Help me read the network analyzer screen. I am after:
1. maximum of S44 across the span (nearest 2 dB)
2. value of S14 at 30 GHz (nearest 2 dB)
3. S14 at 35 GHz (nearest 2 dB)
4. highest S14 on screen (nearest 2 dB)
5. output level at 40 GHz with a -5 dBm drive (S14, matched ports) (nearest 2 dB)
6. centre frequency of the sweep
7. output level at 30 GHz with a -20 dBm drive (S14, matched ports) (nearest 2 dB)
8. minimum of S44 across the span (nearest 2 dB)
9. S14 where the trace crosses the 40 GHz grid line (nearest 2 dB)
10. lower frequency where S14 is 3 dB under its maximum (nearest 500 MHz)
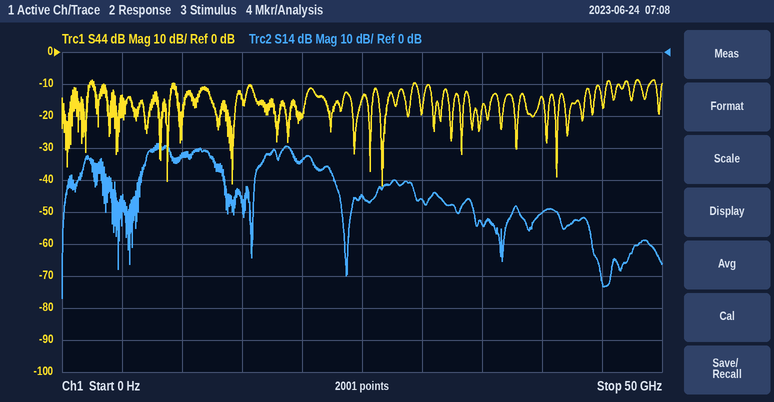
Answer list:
-8 dB
-46 dB
-54 dB
-28 dB
-56 dBm
25 GHz
-66 dBm
-42 dB
-50 dB
7.0 GHz
